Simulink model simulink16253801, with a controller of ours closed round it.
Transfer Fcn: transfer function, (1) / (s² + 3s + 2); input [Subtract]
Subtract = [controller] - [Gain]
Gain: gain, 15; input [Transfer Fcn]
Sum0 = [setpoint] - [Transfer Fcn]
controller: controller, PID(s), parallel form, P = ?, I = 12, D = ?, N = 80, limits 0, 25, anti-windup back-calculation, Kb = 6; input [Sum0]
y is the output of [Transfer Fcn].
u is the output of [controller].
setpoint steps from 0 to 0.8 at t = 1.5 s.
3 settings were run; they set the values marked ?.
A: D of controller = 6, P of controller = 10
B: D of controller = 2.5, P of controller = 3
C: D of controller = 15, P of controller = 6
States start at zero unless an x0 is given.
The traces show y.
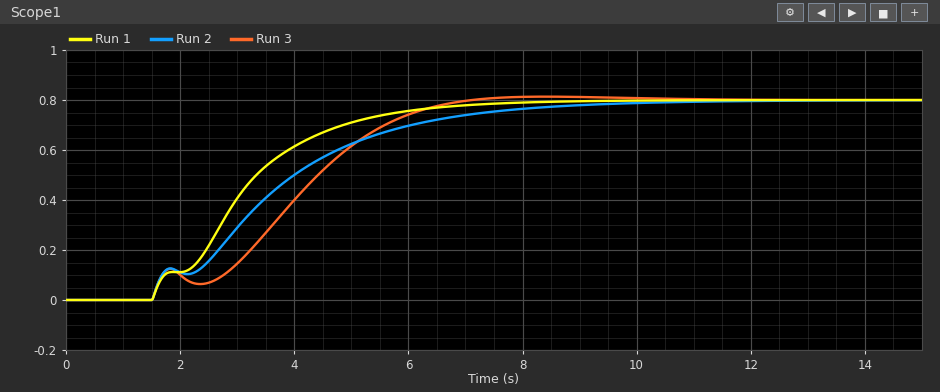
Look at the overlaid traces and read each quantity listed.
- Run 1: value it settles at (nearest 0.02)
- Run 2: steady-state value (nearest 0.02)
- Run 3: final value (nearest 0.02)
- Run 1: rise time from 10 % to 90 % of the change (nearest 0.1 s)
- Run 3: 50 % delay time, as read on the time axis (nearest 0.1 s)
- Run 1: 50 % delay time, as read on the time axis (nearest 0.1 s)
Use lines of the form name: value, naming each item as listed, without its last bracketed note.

Run 1: value it settles at: 0.80
Run 2: steady-state value: 0.80
Run 3: final value: 0.80
Run 1: rise time from 10 % to 90 % of the change: 3.5 s
Run 3: 50 % delay time, as read on the time axis: 4.0 s
Run 1: 50 % delay time, as read on the time axis: 3.0 s
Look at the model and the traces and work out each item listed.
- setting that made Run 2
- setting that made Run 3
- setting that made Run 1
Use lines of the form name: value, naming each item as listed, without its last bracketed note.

setting that made Run 2: A
setting that made Run 3: C
setting that made Run 1: B
